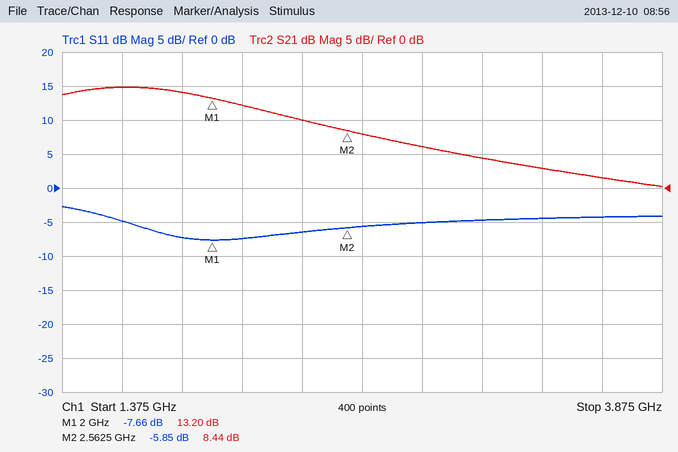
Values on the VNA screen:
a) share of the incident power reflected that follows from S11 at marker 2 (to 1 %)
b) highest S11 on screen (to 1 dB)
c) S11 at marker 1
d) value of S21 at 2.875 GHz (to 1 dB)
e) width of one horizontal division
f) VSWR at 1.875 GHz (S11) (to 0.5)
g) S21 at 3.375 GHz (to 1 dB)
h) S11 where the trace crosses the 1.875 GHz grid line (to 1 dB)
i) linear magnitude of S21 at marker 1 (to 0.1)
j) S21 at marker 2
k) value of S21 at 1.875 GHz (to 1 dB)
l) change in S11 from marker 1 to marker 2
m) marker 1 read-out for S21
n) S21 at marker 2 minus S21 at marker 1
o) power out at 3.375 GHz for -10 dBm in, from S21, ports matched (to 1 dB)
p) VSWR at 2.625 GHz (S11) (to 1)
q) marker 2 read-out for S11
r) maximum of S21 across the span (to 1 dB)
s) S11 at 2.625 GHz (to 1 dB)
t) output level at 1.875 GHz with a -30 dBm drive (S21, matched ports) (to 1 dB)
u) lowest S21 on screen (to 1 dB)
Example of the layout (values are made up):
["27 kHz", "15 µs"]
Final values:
["26 %", "-3 dB", "-7.66 dB", "6 dB", "250 MHz", "2.5", "3 dB", "-7 dB", "4.6", "8.44 dB", "14 dB", "1.81 dB", "13.20 dB", "-4.76 dB", "-7 dBm", "3", "-5.85 dB", "15 dB", "-6 dB", "-16 dBm", "0 dB"]
